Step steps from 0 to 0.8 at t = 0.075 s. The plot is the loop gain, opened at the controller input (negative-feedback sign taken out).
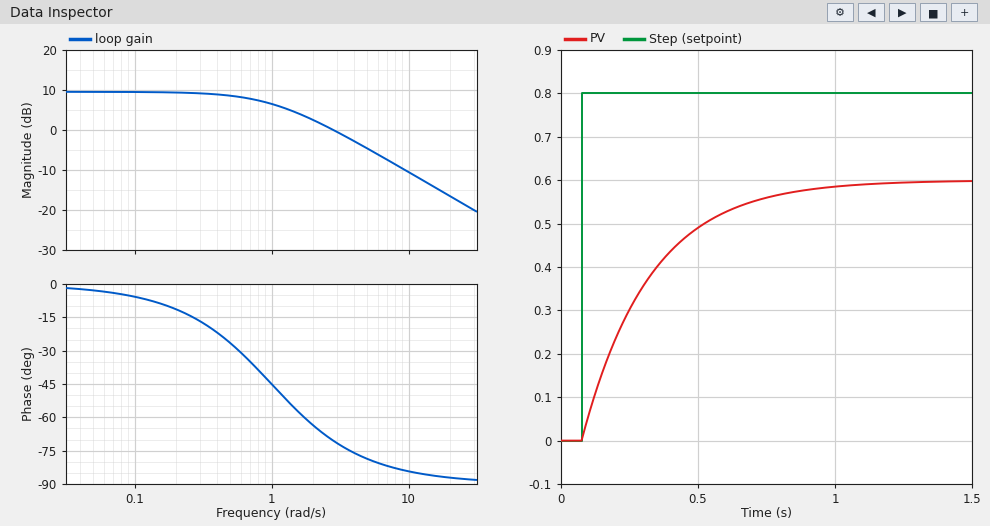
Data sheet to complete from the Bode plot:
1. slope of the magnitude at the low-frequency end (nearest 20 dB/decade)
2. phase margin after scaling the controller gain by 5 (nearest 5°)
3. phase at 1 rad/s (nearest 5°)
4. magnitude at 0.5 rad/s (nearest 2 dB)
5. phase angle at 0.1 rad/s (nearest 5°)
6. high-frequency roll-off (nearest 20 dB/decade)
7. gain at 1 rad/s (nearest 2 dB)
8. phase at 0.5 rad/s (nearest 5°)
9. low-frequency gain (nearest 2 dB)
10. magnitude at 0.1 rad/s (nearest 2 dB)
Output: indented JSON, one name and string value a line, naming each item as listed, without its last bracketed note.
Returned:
{
  "slope of the magnitude at the low-frequency end": "0 dB/decade",
  "phase margin after scaling the controller gain by 5": "95°",
  "phase at 1 rad/s": "-45°",
  "magnitude at 0.5 rad/s": "8 dB",
  "phase angle at 0.1 rad/s": "-5°",
  "high-frequency roll-off": "-20 dB/decade",
  "gain at 1 rad/s": "6 dB",
  "phase at 0.5 rad/s": "-25°",
  "low-frequency gain": "10 dB",
  "magnitude at 0.1 rad/s": "10 dB"
}
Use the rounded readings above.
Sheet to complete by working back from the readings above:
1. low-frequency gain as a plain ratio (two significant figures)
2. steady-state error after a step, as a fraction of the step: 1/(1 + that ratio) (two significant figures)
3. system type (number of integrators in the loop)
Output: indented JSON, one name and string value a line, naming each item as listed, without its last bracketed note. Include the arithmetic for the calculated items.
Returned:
{
  "low-frequency gain as a plain ratio": "10^(10 / 20) = 3.2",
  "steady-state error after a step, as a fraction of the step: 1/(1 + that ratio)": "1 / (1 + 3.2) = 0.24",
  "system type": "0"
}
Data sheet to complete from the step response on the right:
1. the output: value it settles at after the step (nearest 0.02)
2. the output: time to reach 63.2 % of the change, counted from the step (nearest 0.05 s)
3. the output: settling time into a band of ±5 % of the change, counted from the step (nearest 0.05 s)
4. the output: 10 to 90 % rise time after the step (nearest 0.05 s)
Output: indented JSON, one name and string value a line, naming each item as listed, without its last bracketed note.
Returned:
{
  "the output: value it settles at after the step": "0.60",
  "the output: time to reach 63.2 % of the change, counted from the step": "0.25 s",
  "the output: settling time into a band of ±5 % of the change, counted from the step": "0.75 s",
  "the output: 10 to 90 % rise time after the step": "0.55 s"
}
